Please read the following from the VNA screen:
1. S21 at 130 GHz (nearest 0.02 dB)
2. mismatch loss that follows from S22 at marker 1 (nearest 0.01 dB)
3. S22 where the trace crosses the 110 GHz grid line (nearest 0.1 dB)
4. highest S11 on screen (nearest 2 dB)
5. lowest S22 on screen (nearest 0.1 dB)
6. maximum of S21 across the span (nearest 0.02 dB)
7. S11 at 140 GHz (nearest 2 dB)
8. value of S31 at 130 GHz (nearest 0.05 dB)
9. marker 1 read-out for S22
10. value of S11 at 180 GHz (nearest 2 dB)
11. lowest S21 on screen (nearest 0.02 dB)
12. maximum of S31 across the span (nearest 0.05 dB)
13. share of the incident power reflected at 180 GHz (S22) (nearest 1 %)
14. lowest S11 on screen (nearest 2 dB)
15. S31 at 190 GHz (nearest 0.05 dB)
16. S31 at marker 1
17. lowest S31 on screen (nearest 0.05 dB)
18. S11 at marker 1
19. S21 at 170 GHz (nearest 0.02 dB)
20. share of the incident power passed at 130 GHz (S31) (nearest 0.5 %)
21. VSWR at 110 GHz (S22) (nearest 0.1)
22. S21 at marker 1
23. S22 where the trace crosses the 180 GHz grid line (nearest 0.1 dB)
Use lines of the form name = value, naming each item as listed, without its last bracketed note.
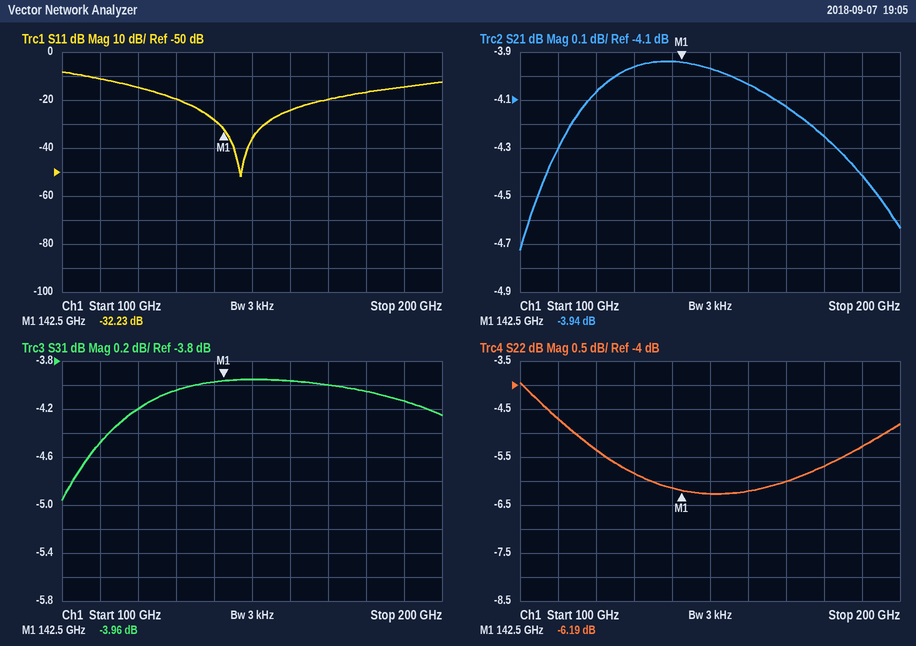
S21 at 130 GHz = -3.96 dB
mismatch loss that follows from S22 at marker 1 = 1.19 dB
S22 where the trace crosses the 110 GHz grid line = -4.7 dB
highest S11 on screen = -8 dB
lowest S22 on screen = -6.3 dB
maximum of S21 across the span = -3.94 dB
S11 at 140 GHz = -28 dB
value of S31 at 130 GHz = -4.05 dB
marker 1 read-out for S22 = -6.19 dB
value of S11 at 180 GHz = -16 dB
lowest S21 on screen = -4.72 dB
maximum of S31 across the span = -3.95 dB
share of the incident power reflected at 180 GHz (S22) = 27 %
lowest S11 on screen = -52 dB
S31 at 190 GHz = -4.15 dB
S31 at marker 1 = -3.96 dB
lowest S31 on screen = -4.95 dB
S11 at marker 1 = -32.23 dB
S21 at 170 GHz = -4.12 dB
share of the incident power passed at 130 GHz (S31) = 39.5 %
VSWR at 110 GHz (S22) = 3.8
S21 at marker 1 = -3.94 dB
S22 where the trace crosses the 180 GHz grid line = -5.7 dB
